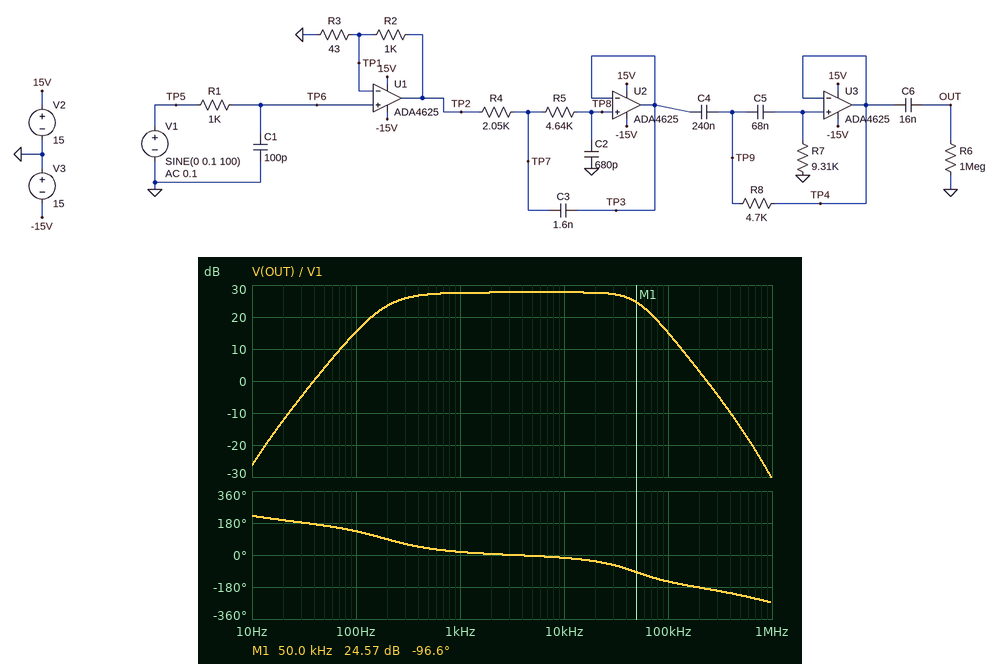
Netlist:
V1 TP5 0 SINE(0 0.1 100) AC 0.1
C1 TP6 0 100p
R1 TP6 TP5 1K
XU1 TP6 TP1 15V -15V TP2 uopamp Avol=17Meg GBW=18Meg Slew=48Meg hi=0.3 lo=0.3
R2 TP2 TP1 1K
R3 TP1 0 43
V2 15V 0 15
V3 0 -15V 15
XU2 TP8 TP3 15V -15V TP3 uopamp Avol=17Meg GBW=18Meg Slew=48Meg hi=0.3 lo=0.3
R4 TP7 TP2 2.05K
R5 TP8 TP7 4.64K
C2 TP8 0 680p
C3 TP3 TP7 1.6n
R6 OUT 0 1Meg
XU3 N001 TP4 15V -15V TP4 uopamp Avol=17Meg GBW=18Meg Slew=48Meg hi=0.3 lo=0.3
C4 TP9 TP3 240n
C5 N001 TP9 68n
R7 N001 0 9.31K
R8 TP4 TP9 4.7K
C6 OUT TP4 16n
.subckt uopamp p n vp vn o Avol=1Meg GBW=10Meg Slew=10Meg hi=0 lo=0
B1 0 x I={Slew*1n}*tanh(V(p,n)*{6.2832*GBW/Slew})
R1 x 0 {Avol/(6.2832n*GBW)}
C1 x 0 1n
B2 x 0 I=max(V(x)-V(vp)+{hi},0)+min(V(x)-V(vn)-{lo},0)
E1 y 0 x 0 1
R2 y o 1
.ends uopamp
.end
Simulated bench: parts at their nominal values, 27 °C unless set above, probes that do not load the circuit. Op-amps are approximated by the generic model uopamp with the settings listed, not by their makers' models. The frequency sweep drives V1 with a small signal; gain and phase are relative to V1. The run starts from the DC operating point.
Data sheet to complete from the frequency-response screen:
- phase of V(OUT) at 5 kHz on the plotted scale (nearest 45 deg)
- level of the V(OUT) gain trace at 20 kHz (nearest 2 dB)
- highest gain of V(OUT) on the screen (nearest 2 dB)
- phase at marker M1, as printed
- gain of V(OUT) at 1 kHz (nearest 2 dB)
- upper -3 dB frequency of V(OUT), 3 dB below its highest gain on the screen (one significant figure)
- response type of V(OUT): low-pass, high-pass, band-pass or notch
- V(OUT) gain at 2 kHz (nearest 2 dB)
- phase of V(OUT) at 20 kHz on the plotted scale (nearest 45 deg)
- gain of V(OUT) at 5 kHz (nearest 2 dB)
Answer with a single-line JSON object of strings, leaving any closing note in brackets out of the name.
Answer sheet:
{"phase of V(OUT) at 5 kHz on the plotted scale": "0 deg", "level of the V(OUT) gain trace at 20 kHz": "28 dB", "highest gain of V(OUT) on the screen": "28 dB", "phase at marker M1, as printed": "-96.6 deg", "gain of V(OUT) at 1 kHz": "28 dB", "upper -3 dB frequency of V(OUT), 3 dB below its highest gain on the screen": "50 kHz", "response type of V(OUT): low-pass, high-pass, band-pass or notch": "band-pass", "V(OUT) gain at 2 kHz": "28 dB", "phase of V(OUT) at 20 kHz on the plotted scale": "-45 deg", "gain of V(OUT) at 5 kHz": "28 dB"}
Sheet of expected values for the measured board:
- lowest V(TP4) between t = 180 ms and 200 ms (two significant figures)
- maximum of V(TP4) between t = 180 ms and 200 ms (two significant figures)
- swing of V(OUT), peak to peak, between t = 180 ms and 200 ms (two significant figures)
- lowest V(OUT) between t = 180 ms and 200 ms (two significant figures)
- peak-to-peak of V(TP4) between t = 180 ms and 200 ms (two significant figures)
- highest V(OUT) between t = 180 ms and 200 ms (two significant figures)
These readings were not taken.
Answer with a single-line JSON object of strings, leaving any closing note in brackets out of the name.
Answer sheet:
{"lowest V(TP4) between t = 180 ms and 200 ms": "-590 mV", "maximum of V(TP4) between t = 180 ms and 200 ms": "590 mV", "swing of V(OUT), peak to peak, between t = 180 ms and 200 ms": "1.2 V", "lowest V(OUT) between t = 180 ms and 200 ms": "-590 mV", "peak-to-peak of V(TP4) between t = 180 ms and 200 ms": "1.2 V", "highest V(OUT) between t = 180 ms and 200 ms": "590 mV"}
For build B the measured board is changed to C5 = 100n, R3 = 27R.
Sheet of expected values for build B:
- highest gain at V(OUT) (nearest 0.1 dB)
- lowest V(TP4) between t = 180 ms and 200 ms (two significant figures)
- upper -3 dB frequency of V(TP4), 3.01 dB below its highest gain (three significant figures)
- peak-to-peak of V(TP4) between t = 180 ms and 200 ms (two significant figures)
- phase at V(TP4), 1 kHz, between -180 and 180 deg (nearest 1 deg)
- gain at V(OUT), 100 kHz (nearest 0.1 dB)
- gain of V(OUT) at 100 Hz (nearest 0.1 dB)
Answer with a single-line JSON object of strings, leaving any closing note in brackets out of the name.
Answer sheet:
{"highest gain at V(OUT)": "31.6 dB", "lowest V(TP4) between t = 180 ms and 200 ms": "-1.4 V", "upper -3 dB frequency of V(TP4), 3.01 dB below its highest gain": "49.2 kHz", "peak-to-peak of V(TP4) between t = 180 ms and 200 ms": "2.7 V", "phase at V(TP4), 1 kHz, between -180 and 180 deg": "12 deg", "gain at V(OUT), 100 kHz": "18.9 dB", "gain of V(OUT) at 100 Hz": "22.6 dB"}
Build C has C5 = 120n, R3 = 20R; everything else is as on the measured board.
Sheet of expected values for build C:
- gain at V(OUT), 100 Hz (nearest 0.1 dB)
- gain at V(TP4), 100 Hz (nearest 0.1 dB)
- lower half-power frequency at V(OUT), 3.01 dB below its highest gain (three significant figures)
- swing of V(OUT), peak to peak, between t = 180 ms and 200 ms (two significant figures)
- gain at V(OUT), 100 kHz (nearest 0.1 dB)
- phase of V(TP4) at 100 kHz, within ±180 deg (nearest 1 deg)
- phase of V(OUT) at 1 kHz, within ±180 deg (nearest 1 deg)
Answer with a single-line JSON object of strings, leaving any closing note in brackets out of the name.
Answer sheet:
{"gain at V(OUT), 100 Hz": "26.6 dB", "gain at V(TP4), 100 Hz": "26.7 dB", "lower half-power frequency at V(OUT), 3.01 dB below its highest gain": "152 Hz", "swing of V(OUT), peak to peak, between t = 180 ms and 200 ms": "4.3 V", "gain at V(OUT), 100 kHz": "21.3 dB", "phase of V(TP4) at 100 kHz, within ±180 deg": "-157 deg", "phase of V(OUT) at 1 kHz, within ±180 deg": "11 deg"}
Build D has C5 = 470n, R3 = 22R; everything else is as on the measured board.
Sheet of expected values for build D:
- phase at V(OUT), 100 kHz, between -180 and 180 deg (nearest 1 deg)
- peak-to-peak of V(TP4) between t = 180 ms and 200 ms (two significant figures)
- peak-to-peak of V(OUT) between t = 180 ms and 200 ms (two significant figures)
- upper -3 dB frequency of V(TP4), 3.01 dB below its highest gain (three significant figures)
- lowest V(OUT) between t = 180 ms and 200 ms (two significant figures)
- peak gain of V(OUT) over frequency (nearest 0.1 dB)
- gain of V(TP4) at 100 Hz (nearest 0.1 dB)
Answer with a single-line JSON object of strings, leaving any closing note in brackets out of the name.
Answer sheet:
{"phase at V(OUT), 100 kHz, between -180 and 180 deg": "-156 deg", "peak-to-peak of V(TP4) between t = 180 ms and 200 ms": "7.9 V", "peak-to-peak of V(OUT) between t = 180 ms and 200 ms": "7.8 V", "upper -3 dB frequency of V(TP4), 3.01 dB below its highest gain": "49.1 kHz", "lowest V(OUT) between t = 180 ms and 200 ms": "-3.9 V", "peak gain of V(OUT) over frequency": "33.3 dB", "gain of V(TP4) at 100 Hz": "31.9 dB"}
